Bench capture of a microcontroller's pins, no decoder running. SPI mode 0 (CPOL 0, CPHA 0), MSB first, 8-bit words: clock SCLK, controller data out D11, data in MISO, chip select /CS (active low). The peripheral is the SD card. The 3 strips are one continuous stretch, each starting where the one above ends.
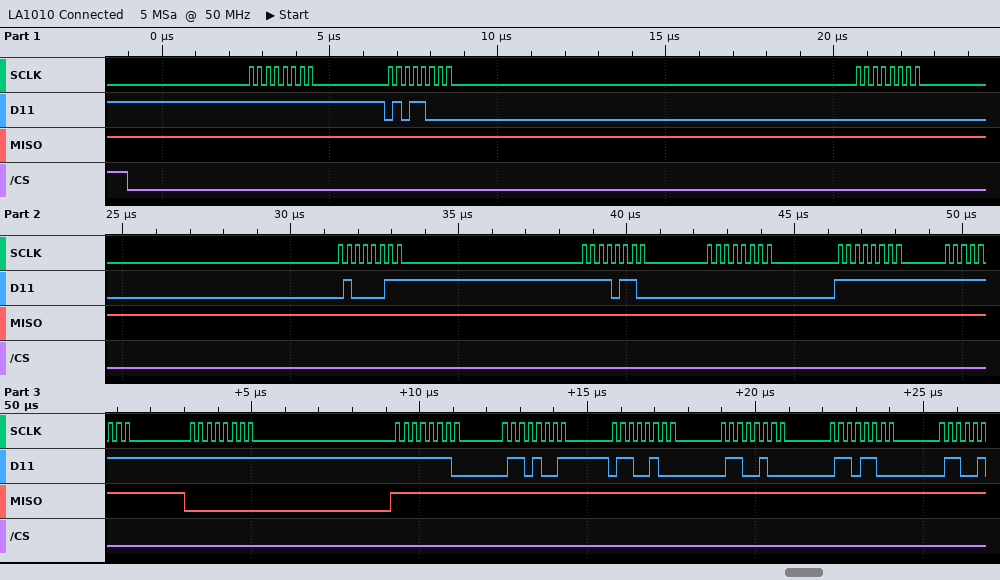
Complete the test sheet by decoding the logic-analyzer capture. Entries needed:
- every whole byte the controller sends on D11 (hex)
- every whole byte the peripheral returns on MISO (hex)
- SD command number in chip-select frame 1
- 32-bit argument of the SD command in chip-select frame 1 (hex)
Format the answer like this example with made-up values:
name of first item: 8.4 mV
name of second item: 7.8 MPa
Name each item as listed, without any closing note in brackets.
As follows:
every whole byte the controller sends on D11: FF 58 00 43 F6 00 FF FF FF FE 69 64 64 6C
every whole byte the peripheral returns on MISO: FF FF FF FF FF FF FF FF 00 FF FF FF FF FF
SD command number in chip-select frame 1: CMD24
32-bit argument of the SD command in chip-select frame 1: 0x0043F600
